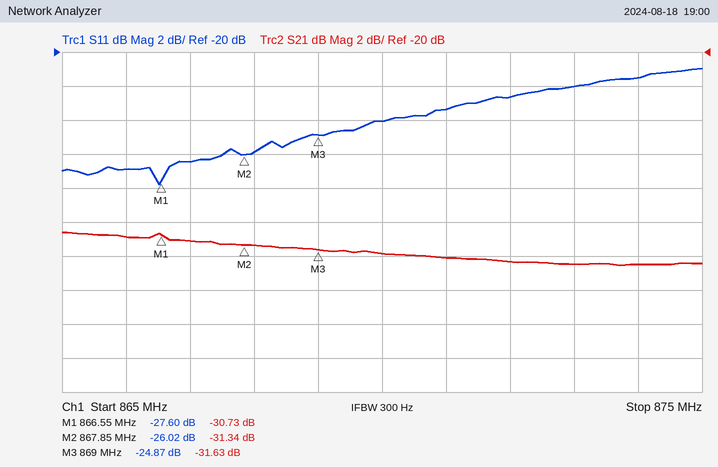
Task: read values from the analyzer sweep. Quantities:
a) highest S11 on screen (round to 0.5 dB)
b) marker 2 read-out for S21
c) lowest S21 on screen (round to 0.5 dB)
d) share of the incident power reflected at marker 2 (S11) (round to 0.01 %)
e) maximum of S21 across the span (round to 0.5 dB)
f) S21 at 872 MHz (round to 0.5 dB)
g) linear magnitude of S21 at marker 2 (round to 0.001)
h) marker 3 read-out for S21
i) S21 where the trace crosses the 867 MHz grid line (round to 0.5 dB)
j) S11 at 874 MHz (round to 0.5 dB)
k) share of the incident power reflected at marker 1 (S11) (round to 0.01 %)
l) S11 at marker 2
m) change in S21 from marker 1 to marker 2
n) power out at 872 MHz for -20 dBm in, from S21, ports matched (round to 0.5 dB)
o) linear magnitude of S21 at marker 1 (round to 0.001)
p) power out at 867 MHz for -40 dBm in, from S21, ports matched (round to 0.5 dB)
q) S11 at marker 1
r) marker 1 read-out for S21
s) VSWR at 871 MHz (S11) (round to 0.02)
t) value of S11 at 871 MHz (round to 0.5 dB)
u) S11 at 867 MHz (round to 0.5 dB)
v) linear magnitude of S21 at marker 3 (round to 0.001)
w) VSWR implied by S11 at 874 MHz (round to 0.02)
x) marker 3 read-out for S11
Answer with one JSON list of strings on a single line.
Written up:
["-21.0 dB", "-31.34 dB", "-32.5 dB", "0.25 %", "-30.5 dB", "-32.5 dB", "0.027", "-31.63 dB", "-31.0 dB", "-21.5 dB", "0.17 %", "-26.02 dB", "-0.61 dB", "-52.5 dBm", "0.029", "-71.0 dBm", "-27.60 dB", "-30.73 dB", "1.14", "-23.5 dB", "-26.5 dB", "0.026", "1.18", "-24.87 dB"]
